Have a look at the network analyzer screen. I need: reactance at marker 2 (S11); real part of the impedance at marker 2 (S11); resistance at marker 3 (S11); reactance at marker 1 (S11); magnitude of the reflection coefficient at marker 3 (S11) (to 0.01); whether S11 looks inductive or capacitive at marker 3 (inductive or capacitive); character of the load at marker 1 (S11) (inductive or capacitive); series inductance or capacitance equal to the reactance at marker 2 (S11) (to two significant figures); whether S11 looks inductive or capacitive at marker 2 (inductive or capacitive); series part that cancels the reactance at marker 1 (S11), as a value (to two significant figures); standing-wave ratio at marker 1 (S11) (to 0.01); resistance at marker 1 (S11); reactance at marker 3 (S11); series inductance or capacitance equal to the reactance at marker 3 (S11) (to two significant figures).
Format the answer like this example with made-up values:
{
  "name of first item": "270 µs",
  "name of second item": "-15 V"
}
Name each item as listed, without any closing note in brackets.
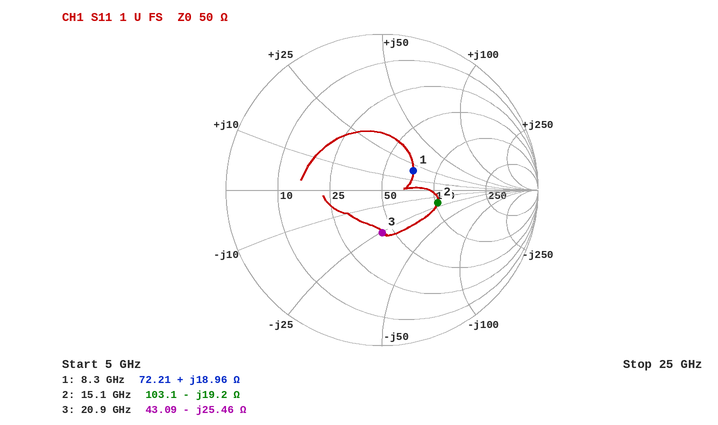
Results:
{
  "reactance at marker 2": "-19.2 Ω",
  "real part of the impedance at marker 2": "103.1 Ω",
  "resistance at marker 3": "43.09 Ω",
  "reactance at marker 1": "+18.96 Ω",
  "magnitude of the reflection coefficient at marker 3 (S11)": "0.27",
  "whether S11 looks inductive or capacitive at marker 3": "capacitive",
  "character of the load at marker 1 (S11)": "inductive",
  "series inductance or capacitance equal to the reactance at marker 2 (S11)": "550 fF",
  "whether S11 looks inductive or capacitive at marker 2": "capacitive",
  "series part that cancels the reactance at marker 1 (S11), as a value": "1.0 pF",
  "standing-wave ratio at marker 1 (S11)": "1.62",
  "resistance at marker 1": "72.21 Ω",
  "reactance at marker 3": "-25.46 Ω",
  "series inductance or capacitance equal to the reactance at marker 3 (S11)": "300 fF"
}
